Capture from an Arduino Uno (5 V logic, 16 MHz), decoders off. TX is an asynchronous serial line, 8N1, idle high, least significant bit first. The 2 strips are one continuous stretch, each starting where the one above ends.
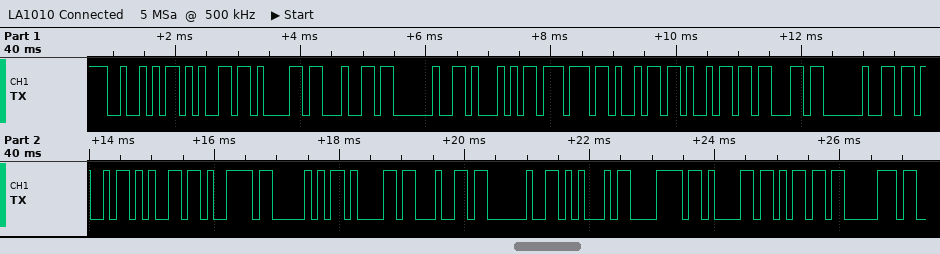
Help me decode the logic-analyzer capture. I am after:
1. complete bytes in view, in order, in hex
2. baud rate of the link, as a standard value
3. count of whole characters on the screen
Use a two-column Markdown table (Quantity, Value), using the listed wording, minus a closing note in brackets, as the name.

| Quantity | Value |
|---|---|
| complete bytes in view, in order, in hex | 52 65 61 64 20 51 77 69 69 63 20 4B 65 79 50 61 64 20 45 78 61 6D 70 |
| baud rate of the link, as a standard value | 9600 baud |
| count of whole characters on the screen | 23 |
